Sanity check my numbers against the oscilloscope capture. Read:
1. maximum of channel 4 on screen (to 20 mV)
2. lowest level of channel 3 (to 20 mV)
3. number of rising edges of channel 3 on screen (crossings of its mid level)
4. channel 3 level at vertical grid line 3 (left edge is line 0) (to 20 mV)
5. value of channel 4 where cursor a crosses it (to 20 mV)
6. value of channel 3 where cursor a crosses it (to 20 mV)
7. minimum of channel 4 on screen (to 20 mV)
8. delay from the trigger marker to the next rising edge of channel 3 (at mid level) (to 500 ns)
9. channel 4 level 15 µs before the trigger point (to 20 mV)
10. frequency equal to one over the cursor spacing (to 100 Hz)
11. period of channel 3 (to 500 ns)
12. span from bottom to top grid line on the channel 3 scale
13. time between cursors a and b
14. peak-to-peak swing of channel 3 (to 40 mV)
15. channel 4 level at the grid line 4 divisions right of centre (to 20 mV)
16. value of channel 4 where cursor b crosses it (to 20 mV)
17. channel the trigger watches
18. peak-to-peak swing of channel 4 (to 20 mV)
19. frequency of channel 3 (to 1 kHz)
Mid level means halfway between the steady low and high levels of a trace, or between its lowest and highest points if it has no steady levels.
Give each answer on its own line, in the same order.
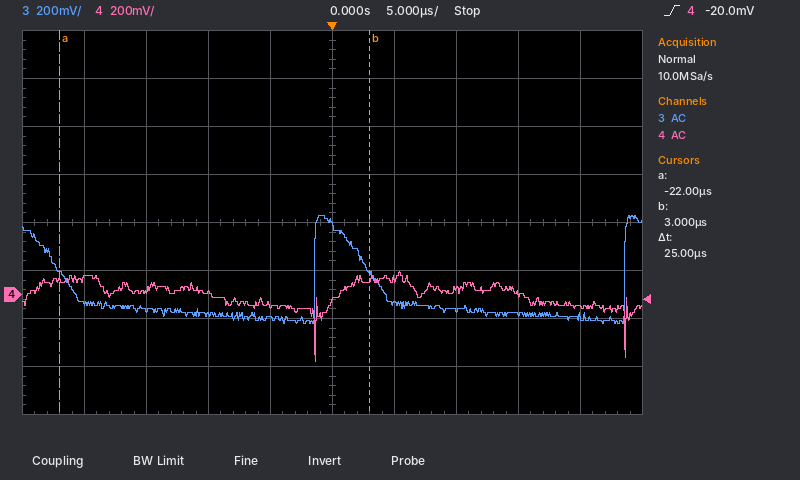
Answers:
100 mV
-120 mV
2
-80 mV
60 mV
100 mV
-280 mV
23.5 µs
20 mV
40.0 kHz
25.0 µs
1.6 V
25 µs
440 mV
-60 mV
60 mV
channel 4
380 mV
40 kHz
